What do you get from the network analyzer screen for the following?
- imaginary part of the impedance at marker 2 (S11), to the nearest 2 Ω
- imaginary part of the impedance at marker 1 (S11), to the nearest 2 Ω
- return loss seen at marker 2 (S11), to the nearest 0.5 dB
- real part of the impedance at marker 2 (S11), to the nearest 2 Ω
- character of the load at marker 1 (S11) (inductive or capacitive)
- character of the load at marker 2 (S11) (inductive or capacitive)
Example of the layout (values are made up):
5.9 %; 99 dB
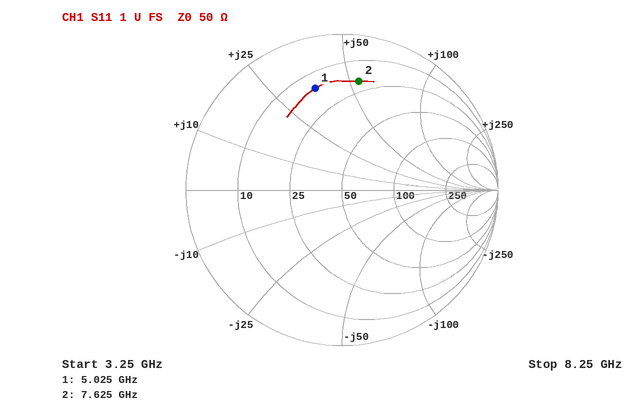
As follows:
+54 Ω; +36 Ω; 3.0 dB; 20 Ω; inductive; inductive
